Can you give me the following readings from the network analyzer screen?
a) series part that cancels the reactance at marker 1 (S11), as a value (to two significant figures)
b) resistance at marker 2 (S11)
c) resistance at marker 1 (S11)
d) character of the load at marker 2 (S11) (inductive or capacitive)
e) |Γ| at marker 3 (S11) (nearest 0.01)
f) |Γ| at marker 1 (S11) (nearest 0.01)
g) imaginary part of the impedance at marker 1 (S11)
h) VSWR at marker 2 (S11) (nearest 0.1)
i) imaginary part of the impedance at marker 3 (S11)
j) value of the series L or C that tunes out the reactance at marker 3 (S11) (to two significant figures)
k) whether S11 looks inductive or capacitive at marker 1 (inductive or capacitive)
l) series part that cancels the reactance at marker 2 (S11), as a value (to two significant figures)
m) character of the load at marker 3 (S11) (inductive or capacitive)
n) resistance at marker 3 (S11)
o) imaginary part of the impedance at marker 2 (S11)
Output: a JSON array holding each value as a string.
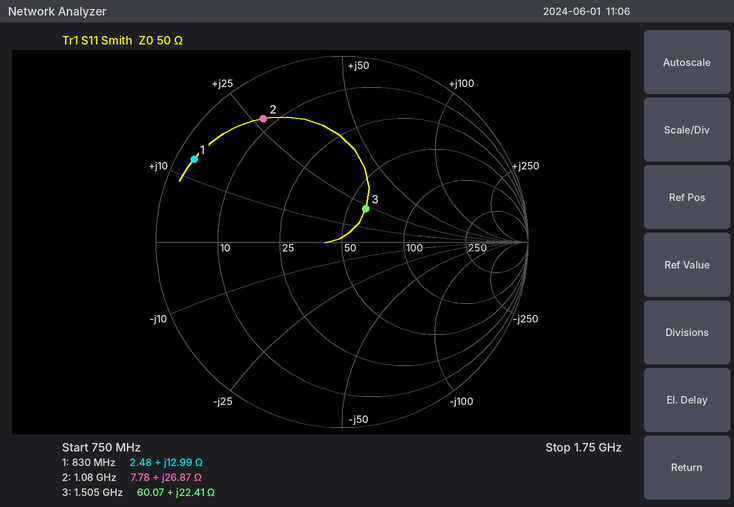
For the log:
["15 pF", "7.78 Ω", "2.48 Ω", "inductive", "0.22", "0.91", "+12.99 Ω", "8.3", "+22.41 Ω", "4.7 pF", "inductive", "5.5 pF", "inductive", "60.07 Ω", "+26.87 Ω"]
